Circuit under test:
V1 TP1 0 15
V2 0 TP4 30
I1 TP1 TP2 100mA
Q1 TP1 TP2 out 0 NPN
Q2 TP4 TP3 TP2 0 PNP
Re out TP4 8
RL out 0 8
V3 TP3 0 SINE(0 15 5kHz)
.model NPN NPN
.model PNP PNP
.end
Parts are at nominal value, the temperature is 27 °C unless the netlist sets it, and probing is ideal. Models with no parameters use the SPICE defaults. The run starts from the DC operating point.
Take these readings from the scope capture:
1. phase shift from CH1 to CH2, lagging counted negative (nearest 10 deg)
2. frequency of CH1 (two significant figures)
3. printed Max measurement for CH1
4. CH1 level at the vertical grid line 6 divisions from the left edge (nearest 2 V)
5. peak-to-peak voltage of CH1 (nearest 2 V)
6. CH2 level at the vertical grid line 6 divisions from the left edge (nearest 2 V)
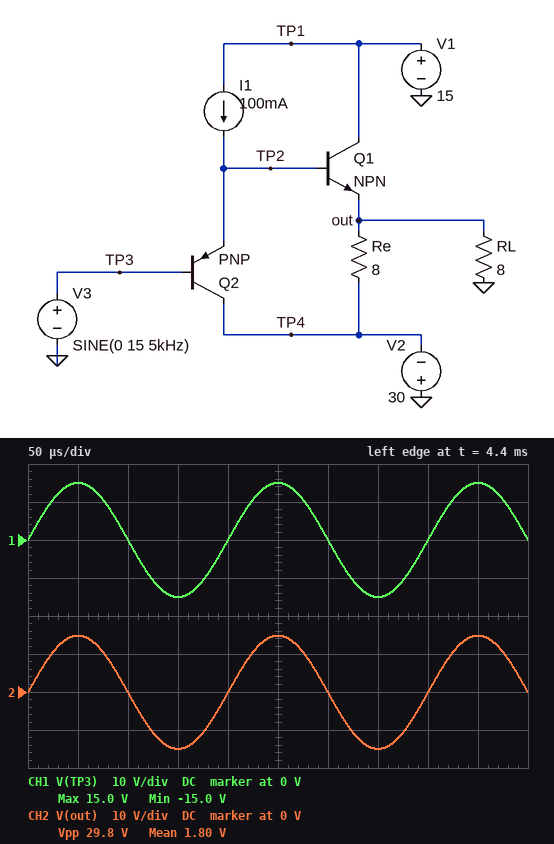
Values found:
0 deg
5.0 kHz
15.0 V
0 V
30 V
0 V
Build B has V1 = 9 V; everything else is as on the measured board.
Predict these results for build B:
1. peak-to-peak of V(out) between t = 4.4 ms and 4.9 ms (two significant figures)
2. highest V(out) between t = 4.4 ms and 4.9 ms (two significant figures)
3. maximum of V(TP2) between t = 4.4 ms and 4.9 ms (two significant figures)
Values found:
24 V
8.9 V
9.9 V
